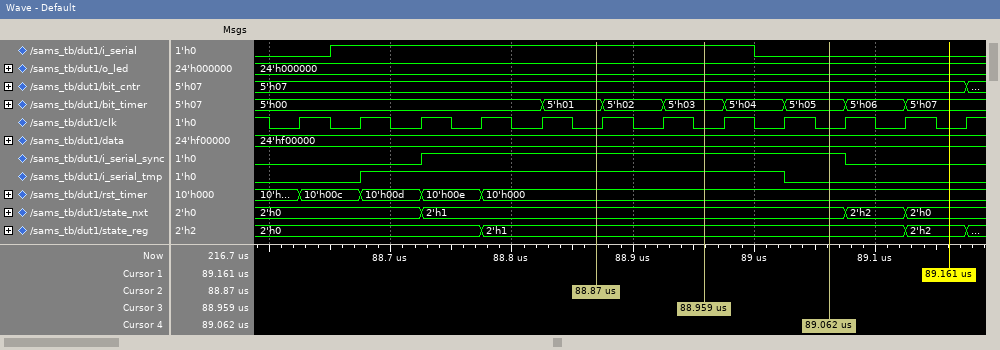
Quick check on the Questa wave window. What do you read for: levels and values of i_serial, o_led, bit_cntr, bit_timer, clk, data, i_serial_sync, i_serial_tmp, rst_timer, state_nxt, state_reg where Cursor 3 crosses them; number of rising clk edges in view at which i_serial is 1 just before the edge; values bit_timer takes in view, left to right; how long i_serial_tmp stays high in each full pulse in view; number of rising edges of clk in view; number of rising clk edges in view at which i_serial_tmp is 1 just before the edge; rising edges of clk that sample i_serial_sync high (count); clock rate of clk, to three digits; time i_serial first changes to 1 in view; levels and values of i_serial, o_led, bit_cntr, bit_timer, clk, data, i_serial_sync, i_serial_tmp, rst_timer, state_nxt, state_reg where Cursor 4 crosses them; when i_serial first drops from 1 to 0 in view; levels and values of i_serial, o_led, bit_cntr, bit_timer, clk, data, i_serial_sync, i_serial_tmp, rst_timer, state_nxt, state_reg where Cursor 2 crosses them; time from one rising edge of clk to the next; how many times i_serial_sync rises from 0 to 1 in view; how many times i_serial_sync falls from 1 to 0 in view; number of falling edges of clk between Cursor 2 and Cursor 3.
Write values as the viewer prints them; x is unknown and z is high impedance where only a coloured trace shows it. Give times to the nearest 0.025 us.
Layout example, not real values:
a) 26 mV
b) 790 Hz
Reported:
a) i_serial=1, o_led=24'h000000, bit_cntr=5'h07, bit_timer=5'h03, clk=0, data=24'hf00000, i_serial_sync=1, i_serial_tmp=1, rst_timer=10'h000, state_nxt=2'h1, state_reg=2'h1
b) 7
c) 5'h00, 5'h01, 5'h02, 5'h03, 5'h04, 5'h05, 5'h06, 5'h07
d) 0.35 us
e) 12
f) 7
g) 7
h) 20.0 MHz
i) 88.65 us
j) i_serial=0, o_led=24'h000000, bit_cntr=5'h07, bit_timer=5'h05, clk=0, data=24'hf00000, i_serial_sync=1, i_serial_tmp=0, rst_timer=10'h000, state_nxt=2'h1, state_reg=2'h1
k) 89 us
l) i_serial=1, o_led=24'h000000, bit_cntr=5'h07, bit_timer=5'h01, clk=0, data=24'hf00000, i_serial_sync=1, i_serial_tmp=1, rst_timer=10'h000, state_nxt=2'h1, state_reg=2'h1
m) 0.05 us
n) 1
o) 1
p) 2
